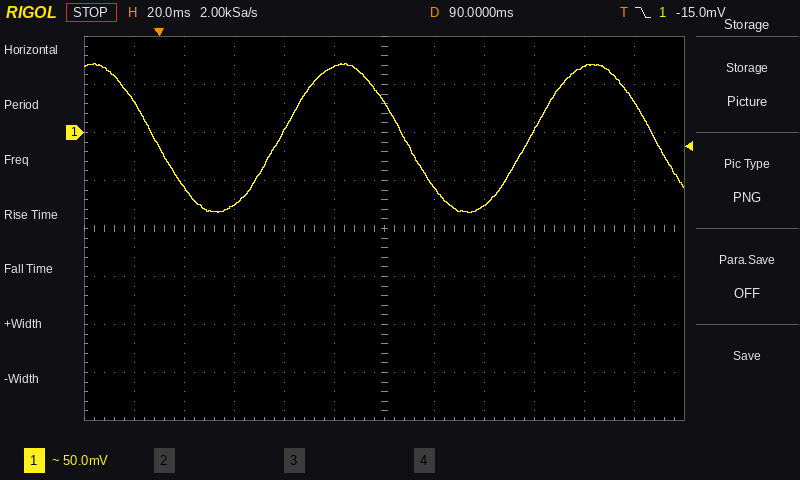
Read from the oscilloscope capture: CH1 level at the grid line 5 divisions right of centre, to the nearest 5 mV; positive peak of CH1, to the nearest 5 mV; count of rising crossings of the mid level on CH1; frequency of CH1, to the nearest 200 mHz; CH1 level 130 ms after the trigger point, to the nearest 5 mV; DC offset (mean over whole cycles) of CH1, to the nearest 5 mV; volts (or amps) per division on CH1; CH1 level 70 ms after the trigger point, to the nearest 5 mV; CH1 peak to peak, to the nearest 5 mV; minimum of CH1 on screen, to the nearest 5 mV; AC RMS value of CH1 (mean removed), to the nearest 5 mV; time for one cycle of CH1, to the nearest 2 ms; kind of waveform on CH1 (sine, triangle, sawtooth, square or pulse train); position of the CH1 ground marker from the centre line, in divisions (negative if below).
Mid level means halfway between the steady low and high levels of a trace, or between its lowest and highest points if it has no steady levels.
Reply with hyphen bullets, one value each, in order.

- 30 mV
- 70 mV
- 2
- 10.0 Hz
- -75 mV
- -5 mV
- 50 mV
- 70 mV
- 155 mV
- -85 mV
- 55 mV
- 100 ms
- sine
- +2.0 div
